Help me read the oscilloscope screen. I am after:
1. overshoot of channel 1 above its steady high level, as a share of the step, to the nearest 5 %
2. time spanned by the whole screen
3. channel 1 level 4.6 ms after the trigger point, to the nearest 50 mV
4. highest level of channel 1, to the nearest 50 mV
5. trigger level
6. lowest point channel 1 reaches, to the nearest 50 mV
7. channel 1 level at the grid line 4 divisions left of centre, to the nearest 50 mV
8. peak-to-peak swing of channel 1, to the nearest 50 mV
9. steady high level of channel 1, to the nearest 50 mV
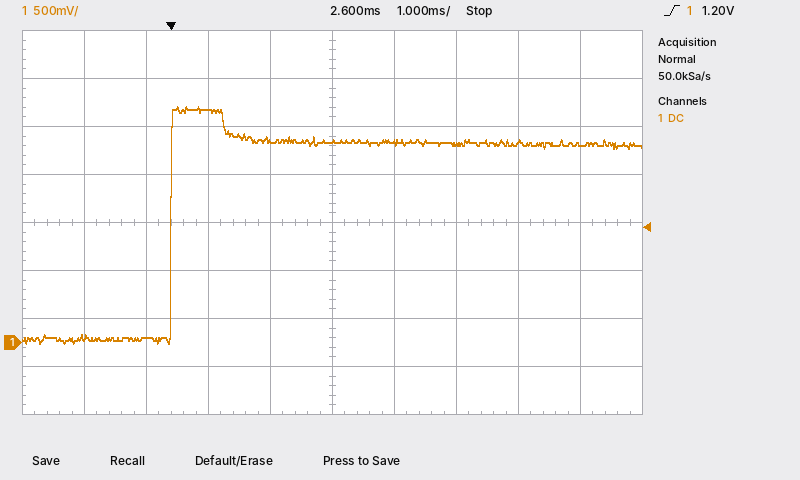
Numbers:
20 %
10 ms
2.05 V
2.45 V
1.20 V
0 mV
50 mV
2.45 V
2.10 V
